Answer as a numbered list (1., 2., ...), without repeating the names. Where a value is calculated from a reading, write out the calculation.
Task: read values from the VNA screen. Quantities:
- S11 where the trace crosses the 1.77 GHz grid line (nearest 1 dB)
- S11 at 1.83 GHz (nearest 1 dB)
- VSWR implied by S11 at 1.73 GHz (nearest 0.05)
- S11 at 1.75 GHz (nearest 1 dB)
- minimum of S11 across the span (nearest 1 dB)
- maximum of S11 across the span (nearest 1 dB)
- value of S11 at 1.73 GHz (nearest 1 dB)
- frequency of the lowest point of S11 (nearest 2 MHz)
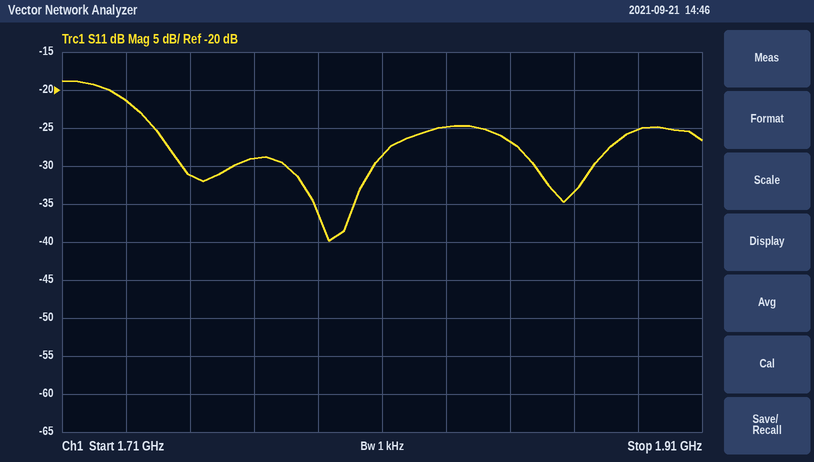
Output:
1. -29 dB
2. -25 dB
3. |Γ| = 10^(-21/20) = 0.0891; VSWR = (1 + 0.0891)/(1 − 0.0891) ≈ 1.20
4. -31 dB
5. -40 dB
6. -19 dB
7. -21 dB
8. 1.794 GHz
